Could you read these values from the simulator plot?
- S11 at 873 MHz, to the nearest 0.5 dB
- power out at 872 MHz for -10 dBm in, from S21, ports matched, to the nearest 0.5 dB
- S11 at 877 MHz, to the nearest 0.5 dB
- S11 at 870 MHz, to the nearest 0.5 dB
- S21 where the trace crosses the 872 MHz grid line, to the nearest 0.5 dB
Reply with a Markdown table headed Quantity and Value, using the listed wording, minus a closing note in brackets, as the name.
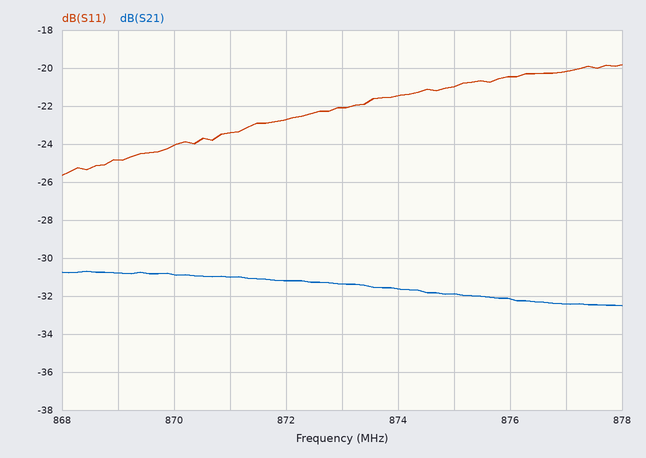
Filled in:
| Quantity | Value |
|---|---|
| S11 at 873 MHz, to the nearest 0.5 dB | -22.0 dB |
| power out at 872 MHz for -10 dBm in, from S21, ports matched, to the nearest 0.5 dB | -41.0 dBm |
| S11 at 877 MHz, to the nearest 0.5 dB | -20.0 dB |
| S11 at 870 MHz, to the nearest 0.5 dB | -24.0 dB |
| S21 where the trace crosses the 872 MHz grid line, to the nearest 0.5 dB | -31.0 dB |
